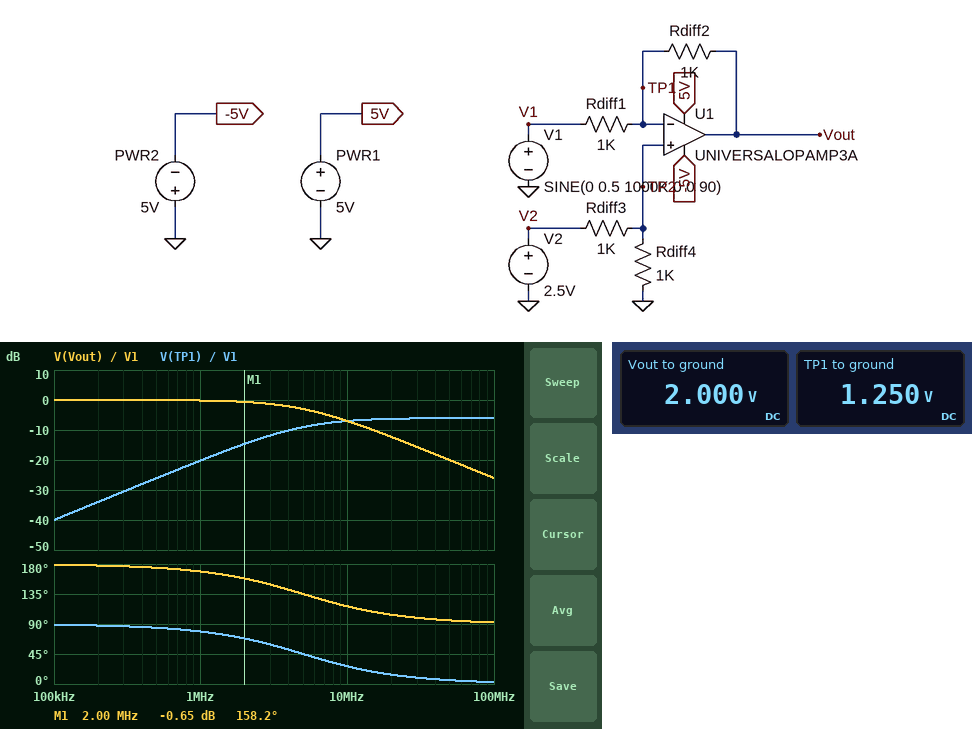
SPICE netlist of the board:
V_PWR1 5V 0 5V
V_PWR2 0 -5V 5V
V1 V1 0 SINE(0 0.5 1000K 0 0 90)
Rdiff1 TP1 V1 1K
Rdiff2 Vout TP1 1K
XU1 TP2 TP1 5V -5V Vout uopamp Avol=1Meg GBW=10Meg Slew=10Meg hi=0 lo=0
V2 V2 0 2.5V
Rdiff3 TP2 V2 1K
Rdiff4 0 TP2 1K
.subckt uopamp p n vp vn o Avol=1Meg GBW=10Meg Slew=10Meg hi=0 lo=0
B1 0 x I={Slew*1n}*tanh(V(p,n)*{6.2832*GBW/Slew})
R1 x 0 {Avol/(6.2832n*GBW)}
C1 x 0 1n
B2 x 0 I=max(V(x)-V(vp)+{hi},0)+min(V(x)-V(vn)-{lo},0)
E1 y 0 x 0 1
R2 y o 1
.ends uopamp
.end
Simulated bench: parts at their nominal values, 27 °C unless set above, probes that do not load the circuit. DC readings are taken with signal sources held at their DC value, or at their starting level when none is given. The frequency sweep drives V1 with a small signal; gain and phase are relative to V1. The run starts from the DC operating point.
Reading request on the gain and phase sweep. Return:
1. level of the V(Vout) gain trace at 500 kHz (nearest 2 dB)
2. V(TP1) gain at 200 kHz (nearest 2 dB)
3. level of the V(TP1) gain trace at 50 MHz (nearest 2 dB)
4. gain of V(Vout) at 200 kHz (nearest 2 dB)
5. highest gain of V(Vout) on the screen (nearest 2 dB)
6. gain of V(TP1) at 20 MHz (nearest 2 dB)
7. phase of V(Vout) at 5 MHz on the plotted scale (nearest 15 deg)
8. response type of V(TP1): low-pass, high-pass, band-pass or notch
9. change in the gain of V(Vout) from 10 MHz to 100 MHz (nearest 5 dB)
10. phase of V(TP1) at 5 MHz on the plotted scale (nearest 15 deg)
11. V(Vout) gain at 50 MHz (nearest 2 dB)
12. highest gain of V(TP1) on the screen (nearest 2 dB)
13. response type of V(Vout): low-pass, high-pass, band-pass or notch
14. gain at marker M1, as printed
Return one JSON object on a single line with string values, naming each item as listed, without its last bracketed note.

{"level of the V(Vout) gain trace at 500 kHz": "0 dB", "V(TP1) gain at 200 kHz": "-34 dB", "level of the V(TP1) gain trace at 50 MHz": "-6 dB", "gain of V(Vout) at 200 kHz": "0 dB", "highest gain of V(Vout) on the screen": "0 dB", "gain of V(TP1) at 20 MHz": "-6 dB", "phase of V(Vout) at 5 MHz on the plotted scale": "135 deg", "response type of V(TP1): low-pass, high-pass, band-pass or notch": "high-pass", "change in the gain of V(Vout) from 10 MHz to 100 MHz": "-20 dB", "phase of V(TP1) at 5 MHz on the plotted scale": "45 deg", "V(Vout) gain at 50 MHz": "-20 dB", "highest gain of V(TP1) on the screen": "-6 dB", "response type of V(Vout): low-pass, high-pass, band-pass or notch": "low-pass", "gain at marker M1, as printed": "-0.65 dB"}
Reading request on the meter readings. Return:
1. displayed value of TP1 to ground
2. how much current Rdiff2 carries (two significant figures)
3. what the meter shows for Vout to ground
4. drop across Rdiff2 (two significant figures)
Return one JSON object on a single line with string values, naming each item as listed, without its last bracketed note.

{"displayed value of TP1 to ground": "1.250 V", "how much current Rdiff2 carries": "750 µA", "what the meter shows for Vout to ground": "2.000 V", "drop across Rdiff2": "750 mV"}
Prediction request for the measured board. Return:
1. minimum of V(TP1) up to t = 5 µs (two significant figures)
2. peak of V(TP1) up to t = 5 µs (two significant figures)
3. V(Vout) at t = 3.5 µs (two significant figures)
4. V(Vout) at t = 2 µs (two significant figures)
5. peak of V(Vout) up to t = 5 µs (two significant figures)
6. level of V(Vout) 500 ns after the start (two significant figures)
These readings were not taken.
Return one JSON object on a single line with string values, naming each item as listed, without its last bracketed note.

{"minimum of V(TP1) up to t = 5 µs": "1.2 V", "peak of V(TP1) up to t = 5 µs": "1.3 V", "V(Vout) at t = 3.5 µs": "3.0 V", "V(Vout) at t = 2 µs": "2.0 V", "peak of V(Vout) up to t = 5 µs": "3.0 V", "level of V(Vout) 500 ns after the start": "3.0 V"}
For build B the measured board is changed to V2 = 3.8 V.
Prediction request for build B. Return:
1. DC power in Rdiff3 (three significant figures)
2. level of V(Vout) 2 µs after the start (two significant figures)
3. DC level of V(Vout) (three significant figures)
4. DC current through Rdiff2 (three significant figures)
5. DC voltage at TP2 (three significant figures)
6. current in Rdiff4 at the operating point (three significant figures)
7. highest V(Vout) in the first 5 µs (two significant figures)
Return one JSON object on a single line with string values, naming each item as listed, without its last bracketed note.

{"DC power in Rdiff3": "3.61 mW", "level of V(Vout) 2 µs after the start": "3.3 V", "DC level of V(Vout)": "3.30 V", "DC current through Rdiff2": "1.40 mA", "DC voltage at TP2": "1.90 V", "current in Rdiff4 at the operating point": "1.90 mA", "highest V(Vout) in the first 5 µs": "4.3 V"}
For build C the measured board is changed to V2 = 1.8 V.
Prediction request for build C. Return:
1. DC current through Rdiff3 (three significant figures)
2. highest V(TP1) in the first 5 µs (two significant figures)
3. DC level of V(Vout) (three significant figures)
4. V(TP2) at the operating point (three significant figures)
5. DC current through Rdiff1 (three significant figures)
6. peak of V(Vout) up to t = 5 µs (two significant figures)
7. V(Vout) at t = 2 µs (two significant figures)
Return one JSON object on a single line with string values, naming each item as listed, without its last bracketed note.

{"DC current through Rdiff3": "900 µA", "highest V(TP1) in the first 5 µs": "950 mV", "DC level of V(Vout)": "1.30 V", "V(TP2) at the operating point": "900 mV", "DC current through Rdiff1": "400 µA", "peak of V(Vout) up to t = 5 µs": "2.3 V", "V(Vout) at t = 2 µs": "1.3 V"}
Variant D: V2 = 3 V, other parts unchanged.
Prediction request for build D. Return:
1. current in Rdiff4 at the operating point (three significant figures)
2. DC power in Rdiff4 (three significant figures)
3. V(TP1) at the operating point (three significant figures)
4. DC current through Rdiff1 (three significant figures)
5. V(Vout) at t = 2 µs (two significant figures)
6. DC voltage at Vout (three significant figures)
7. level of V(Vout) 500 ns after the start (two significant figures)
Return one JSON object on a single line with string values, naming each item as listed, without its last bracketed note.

{"current in Rdiff4 at the operating point": "1.50 mA", "DC power in Rdiff4": "2.25 mW", "V(TP1) at the operating point": "1.50 V", "DC current through Rdiff1": "1.00 mA", "V(Vout) at t = 2 µs": "2.5 V", "DC voltage at Vout": "2.50 V", "level of V(Vout) 500 ns after the start": "3.5 V"}
